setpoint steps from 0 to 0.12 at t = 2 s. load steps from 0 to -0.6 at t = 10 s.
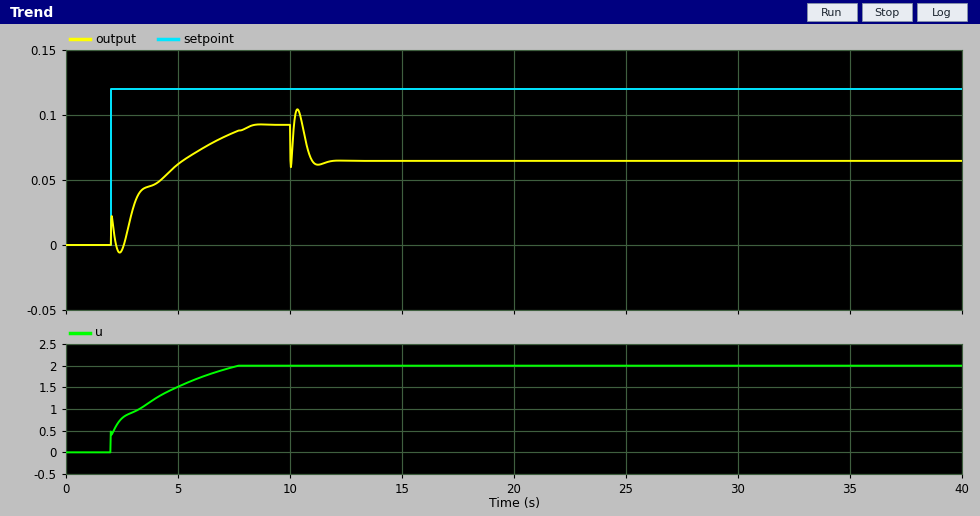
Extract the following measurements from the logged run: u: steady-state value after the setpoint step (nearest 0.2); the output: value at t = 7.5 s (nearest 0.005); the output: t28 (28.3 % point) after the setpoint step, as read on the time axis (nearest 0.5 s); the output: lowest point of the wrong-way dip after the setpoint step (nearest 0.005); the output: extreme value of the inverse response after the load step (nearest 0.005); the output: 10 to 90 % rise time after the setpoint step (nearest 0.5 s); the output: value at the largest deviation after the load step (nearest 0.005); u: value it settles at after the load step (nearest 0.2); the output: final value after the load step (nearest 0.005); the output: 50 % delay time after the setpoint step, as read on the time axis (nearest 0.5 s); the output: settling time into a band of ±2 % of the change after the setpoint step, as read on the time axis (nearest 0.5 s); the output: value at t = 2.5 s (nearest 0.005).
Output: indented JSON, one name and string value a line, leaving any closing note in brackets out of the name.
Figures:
{
  "u: steady-state value after the setpoint step": "2.0",
  "the output: value at t = 7.5 s": "0.085",
  "the output: t28 (28.3 % point) after the setpoint step, as read on the time axis": "3.0 s",
  "the output: lowest point of the wrong-way dip after the setpoint step": "-0.005",
  "the output: extreme value of the inverse response after the load step": "0.105",
  "the output: 10 to 90 % rise time after the setpoint step": "5.0 s",
  "the output: value at the largest deviation after the load step": "0.060",
  "u: value it settles at after the load step": "2.0",
  "the output: final value after the load step": "0.065",
  "the output: 50 % delay time after the setpoint step, as read on the time axis": "4.0 s",
  "the output: settling time into a band of ±2 % of the change after the setpoint step, as read on the time axis": "8.0 s",
  "the output: value at t = 2.5 s": "-0.005"
}
